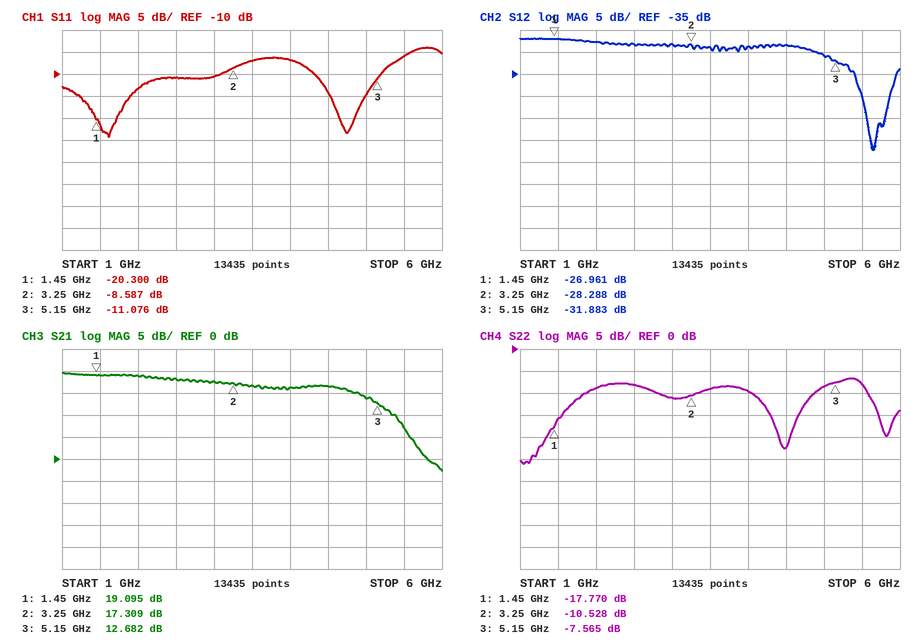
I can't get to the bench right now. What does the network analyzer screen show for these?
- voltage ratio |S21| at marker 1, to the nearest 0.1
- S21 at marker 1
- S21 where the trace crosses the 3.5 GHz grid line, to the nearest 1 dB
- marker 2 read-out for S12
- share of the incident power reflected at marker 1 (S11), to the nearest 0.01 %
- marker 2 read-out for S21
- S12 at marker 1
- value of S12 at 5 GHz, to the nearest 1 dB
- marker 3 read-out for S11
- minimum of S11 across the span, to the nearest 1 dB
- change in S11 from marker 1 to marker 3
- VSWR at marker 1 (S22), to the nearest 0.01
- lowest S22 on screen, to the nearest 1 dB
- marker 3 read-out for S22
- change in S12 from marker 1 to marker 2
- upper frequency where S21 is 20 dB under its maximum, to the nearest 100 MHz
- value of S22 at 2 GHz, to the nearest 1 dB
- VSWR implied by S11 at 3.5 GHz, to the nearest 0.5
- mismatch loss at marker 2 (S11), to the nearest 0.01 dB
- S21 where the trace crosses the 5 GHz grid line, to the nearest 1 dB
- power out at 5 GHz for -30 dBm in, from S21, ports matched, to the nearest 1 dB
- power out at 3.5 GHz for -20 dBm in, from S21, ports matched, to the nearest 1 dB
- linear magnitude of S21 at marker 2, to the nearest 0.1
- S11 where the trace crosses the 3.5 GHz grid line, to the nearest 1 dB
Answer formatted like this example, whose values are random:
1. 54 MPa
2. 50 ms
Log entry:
1. 9.0
2. 19.095 dB
3. 17 dB
4. -28.288 dB
5. 0.93 %
6. 17.309 dB
7. -26.961 dB
8. -31 dB
9. -11.076 dB
10. -24 dB
11. 9.224 dB
12. 1.30
13. -26 dB
14. -7.565 dB
15. -1.327 dB
16. 5.8 GHz
17. -9 dB
18. 2.5
19. 0.65 dB
20. 14 dB
21. -16 dBm
22. -3 dBm
23. 7.3
24. -7 dB
